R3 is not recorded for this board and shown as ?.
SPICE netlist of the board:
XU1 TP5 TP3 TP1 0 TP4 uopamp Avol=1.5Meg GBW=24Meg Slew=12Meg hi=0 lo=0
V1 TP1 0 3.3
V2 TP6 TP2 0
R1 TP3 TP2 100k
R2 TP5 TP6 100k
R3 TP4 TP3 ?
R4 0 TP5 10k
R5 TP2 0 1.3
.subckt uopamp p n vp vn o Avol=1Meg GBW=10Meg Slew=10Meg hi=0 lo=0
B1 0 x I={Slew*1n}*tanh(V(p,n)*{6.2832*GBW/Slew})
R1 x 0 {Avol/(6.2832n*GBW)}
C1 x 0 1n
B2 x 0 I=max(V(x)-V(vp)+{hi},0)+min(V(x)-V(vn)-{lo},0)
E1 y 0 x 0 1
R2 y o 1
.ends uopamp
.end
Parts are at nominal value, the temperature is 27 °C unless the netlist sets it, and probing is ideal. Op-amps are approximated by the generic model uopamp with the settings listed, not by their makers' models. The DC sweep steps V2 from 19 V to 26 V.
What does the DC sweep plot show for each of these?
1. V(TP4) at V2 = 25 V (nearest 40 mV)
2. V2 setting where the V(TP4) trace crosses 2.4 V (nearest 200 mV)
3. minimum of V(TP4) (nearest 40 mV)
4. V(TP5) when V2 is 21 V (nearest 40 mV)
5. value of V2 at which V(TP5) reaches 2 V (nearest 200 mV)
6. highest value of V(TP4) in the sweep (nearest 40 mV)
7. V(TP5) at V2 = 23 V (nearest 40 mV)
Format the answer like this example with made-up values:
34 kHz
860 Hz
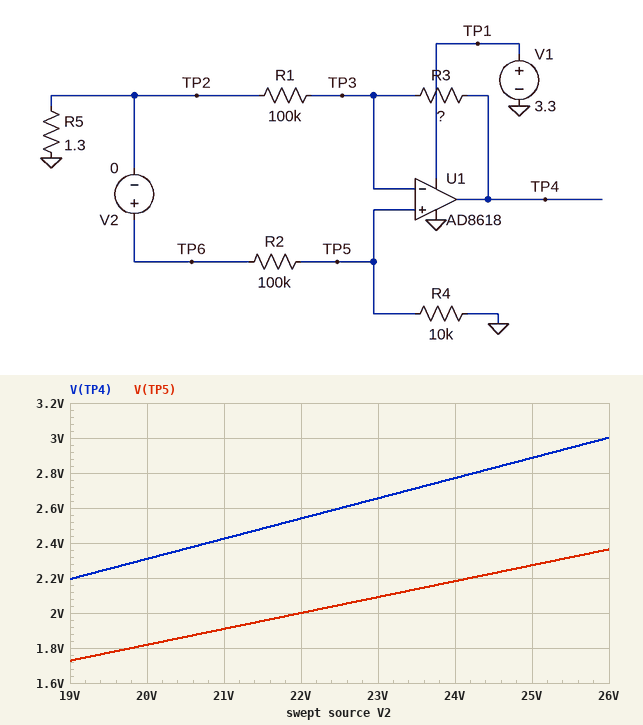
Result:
2.88 V
20.8 V
2.20 V
1.92 V
22.0 V
3.00 V
2.08 V
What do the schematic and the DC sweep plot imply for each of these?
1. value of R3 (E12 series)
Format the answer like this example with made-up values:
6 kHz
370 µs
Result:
27 kΩ
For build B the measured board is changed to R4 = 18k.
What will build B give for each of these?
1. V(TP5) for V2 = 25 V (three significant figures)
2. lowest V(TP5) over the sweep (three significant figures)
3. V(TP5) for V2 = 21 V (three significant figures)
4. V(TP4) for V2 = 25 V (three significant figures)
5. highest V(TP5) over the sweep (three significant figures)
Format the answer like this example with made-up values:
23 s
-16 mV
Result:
3.81 V
2.90 V
3.20 V
3.31 V
3.97 V
